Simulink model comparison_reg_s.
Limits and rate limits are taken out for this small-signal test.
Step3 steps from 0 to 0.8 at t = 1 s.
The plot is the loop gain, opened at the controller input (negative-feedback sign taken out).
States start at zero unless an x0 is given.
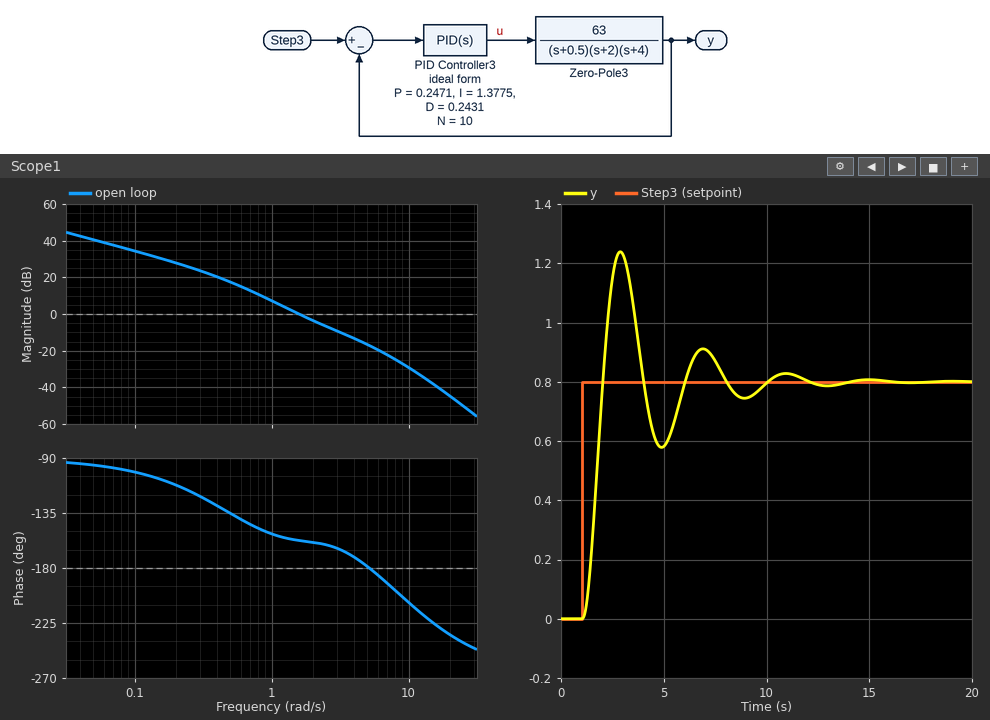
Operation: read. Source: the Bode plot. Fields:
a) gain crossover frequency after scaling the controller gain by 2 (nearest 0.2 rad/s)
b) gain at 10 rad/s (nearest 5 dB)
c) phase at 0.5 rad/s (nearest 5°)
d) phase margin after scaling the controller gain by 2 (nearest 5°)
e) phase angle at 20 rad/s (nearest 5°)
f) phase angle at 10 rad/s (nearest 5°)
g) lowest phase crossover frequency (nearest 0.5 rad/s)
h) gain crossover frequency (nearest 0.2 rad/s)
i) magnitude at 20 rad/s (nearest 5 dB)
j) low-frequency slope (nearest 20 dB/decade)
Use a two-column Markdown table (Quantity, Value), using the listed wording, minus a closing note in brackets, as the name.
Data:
| Quantity | Value |
|---|---|
| gain crossover frequency after scaling the controller gain by 2 | 2.4 rad/s |
| gain at 10 rad/s | -30 dB |
| phase at 0.5 rad/s | -135° |
| phase margin after scaling the controller gain by 2 | 20° |
| phase angle at 20 rad/s | -235° |
| phase angle at 10 rad/s | -210° |
| lowest phase crossover frequency | 5.0 rad/s |
| gain crossover frequency | 1.6 rad/s |
| magnitude at 20 rad/s | -45 dB |
| low-frequency slope | -20 dB/decade |
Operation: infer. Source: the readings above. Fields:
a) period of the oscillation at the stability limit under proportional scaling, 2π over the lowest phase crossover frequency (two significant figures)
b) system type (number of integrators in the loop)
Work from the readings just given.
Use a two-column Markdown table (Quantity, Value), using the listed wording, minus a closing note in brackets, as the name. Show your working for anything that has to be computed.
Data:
| Quantity | Value |
|---|---|
| period of the oscillation at the stability limit under proportional scaling, 2π over the lowest phase crossover frequency | 2π / 5 = 1.3 s |
| system type | 1 |
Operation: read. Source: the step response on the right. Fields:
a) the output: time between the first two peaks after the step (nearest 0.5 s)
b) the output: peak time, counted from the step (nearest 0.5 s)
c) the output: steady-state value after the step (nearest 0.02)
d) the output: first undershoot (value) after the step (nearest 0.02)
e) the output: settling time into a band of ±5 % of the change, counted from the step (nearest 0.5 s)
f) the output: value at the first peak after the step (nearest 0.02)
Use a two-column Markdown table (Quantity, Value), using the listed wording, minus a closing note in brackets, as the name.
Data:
| Quantity | Value |
|---|---|
| the output: time between the first two peaks after the step | 4.0 s |
| the output: peak time, counted from the step | 2.0 s |
| the output: steady-state value after the step | 0.80 |
| the output: first undershoot (value) after the step | 0.58 |
| the output: settling time into a band of ±5 % of the change, counted from the step | 8.5 s |
| the output: value at the first peak after the step | 1.24 |
